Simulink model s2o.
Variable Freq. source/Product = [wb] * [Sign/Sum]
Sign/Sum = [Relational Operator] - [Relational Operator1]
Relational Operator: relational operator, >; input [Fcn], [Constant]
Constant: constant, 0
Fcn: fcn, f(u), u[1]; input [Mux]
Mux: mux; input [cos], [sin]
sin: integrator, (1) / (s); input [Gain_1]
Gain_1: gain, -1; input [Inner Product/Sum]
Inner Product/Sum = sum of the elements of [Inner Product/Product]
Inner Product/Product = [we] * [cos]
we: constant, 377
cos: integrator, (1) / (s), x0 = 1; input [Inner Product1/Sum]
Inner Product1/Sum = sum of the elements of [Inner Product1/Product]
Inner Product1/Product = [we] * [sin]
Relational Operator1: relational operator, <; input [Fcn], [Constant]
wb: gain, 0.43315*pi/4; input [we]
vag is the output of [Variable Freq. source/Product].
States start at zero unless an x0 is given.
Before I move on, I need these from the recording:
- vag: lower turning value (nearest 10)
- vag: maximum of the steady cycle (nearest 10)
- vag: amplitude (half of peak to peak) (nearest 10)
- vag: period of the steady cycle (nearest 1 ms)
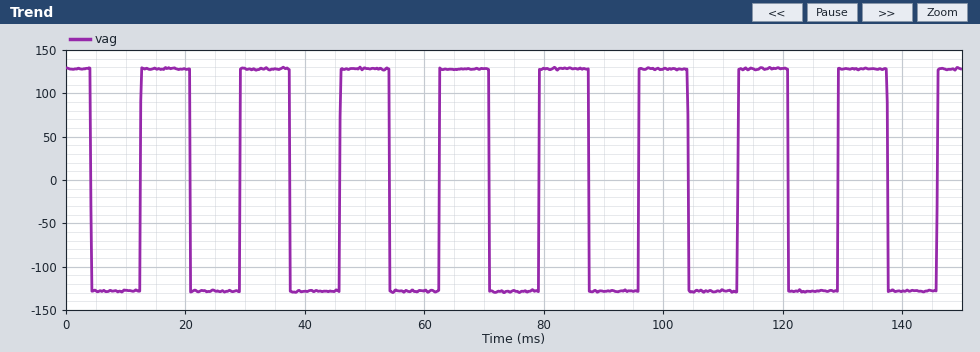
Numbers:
-130
130
130
17 ms
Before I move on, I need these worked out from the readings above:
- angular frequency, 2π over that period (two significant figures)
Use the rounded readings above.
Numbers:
0.37 rad/ms
